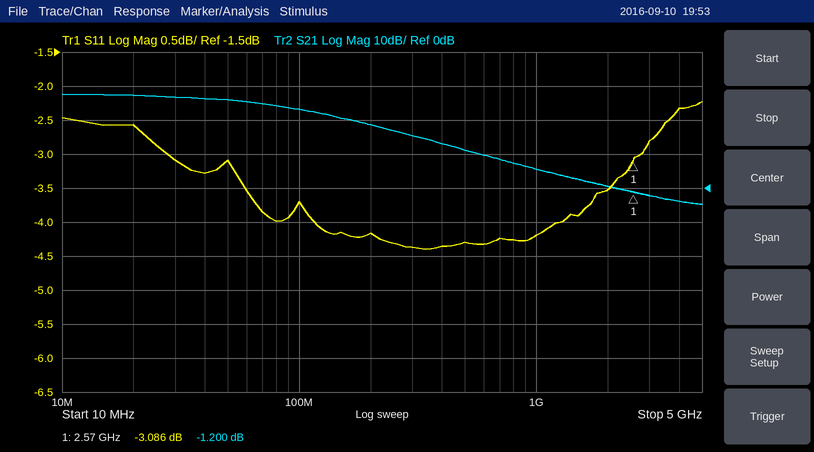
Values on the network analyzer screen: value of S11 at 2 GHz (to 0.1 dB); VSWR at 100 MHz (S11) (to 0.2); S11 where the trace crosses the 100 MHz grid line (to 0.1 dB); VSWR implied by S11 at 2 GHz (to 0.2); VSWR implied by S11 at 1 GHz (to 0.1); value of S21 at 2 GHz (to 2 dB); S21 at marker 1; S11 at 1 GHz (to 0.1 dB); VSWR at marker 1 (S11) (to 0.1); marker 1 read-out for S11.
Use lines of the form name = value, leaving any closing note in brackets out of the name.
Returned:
value of S11 at 2 GHz = -3.5 dB
VSWR at 100 MHz (S11) = 4.8
S11 where the trace crosses the 100 MHz grid line = -3.7 dB
VSWR implied by S11 at 2 GHz = 5.0
VSWR implied by S11 at 1 GHz = 4.2
value of S21 at 2 GHz = 0 dB
S21 at marker 1 = -1.200 dB
S11 at 1 GHz = -4.2 dB
VSWR at marker 1 (S11) = 5.7
marker 1 read-out for S11 = -3.086 dB
